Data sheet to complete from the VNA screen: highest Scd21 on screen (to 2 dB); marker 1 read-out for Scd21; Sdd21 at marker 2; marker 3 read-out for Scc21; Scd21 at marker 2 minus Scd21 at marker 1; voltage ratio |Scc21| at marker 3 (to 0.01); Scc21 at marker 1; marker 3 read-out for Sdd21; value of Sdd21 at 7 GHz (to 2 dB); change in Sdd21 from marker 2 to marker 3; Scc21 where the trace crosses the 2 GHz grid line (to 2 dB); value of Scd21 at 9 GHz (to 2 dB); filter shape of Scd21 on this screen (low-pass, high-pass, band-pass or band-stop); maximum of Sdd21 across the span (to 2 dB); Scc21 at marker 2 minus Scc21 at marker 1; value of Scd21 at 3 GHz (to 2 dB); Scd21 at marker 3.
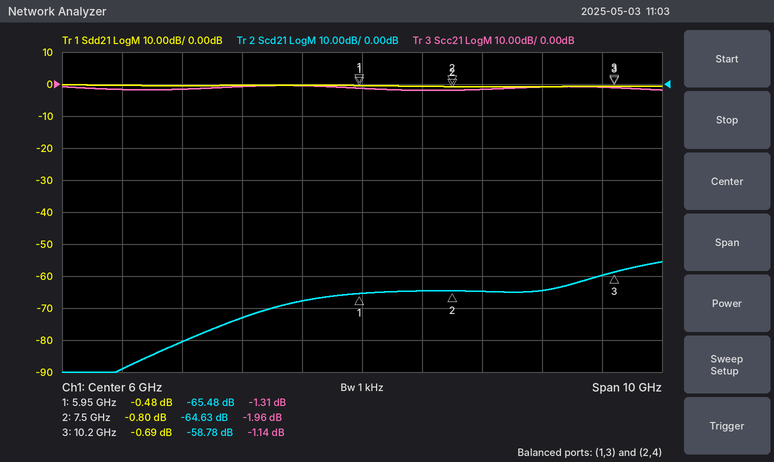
-56 dB
-65.48 dB
-0.80 dB
-1.14 dB
0.85 dB
0.88
-1.31 dB
-0.69 dB
0 dB
0.11 dB
-2 dB
-64 dB
high-pass
0 dB
-0.65 dB
-80 dB
-58.78 dB
